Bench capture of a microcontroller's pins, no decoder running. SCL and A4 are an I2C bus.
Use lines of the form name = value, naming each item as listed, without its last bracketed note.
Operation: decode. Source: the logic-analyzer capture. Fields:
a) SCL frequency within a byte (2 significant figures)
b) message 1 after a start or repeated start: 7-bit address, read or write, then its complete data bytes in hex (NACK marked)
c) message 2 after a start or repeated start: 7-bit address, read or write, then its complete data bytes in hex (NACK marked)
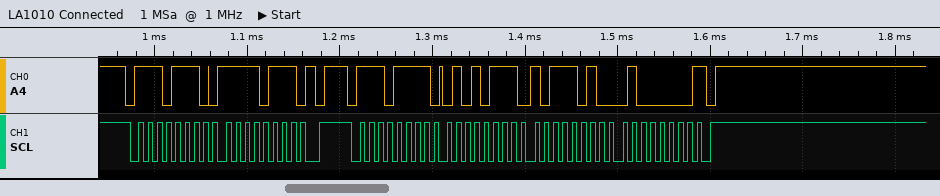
SCL frequency within a byte = 100 kHz
message 1 after a start or repeated start: 7-bit address, read or write, then its complete data bytes in hex = 0x77 write: F7
message 2 after a start or repeated start: 7-bit address, read or write, then its complete data bytes in hex = 0x77 read: 57 BA 40 NACK
